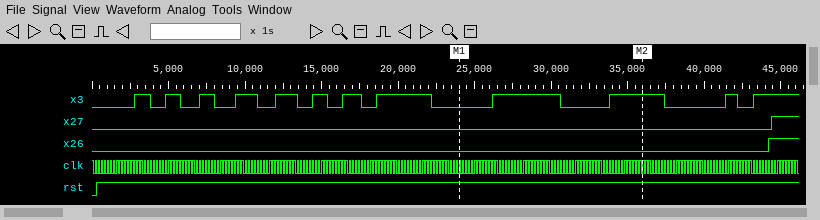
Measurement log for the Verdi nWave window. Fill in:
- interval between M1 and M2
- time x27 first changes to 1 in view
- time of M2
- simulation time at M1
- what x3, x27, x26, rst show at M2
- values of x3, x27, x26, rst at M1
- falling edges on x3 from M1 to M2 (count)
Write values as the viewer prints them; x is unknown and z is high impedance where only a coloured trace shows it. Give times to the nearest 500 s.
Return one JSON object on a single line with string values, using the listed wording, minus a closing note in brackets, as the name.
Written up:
{"interval between M1 and M2": "12000 s", "time x27 first changes to 1 in view": "44500 s", "time of M2": "36000 s", "simulation time at M1": "24000 s", "what x3, x27, x26, rst show at M2": "x3=1, x27=0, x26=0, rst=1", "values of x3, x27, x26, rst at M1": "x3=0, x27=0, x26=0, rst=1", "falling edges on x3 from M1 to M2": "1"}
